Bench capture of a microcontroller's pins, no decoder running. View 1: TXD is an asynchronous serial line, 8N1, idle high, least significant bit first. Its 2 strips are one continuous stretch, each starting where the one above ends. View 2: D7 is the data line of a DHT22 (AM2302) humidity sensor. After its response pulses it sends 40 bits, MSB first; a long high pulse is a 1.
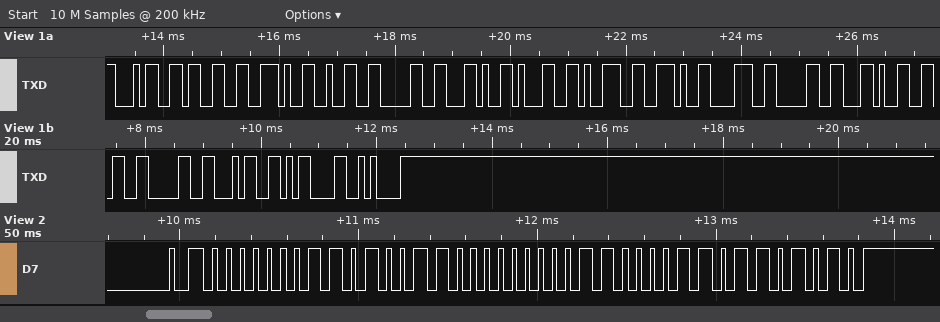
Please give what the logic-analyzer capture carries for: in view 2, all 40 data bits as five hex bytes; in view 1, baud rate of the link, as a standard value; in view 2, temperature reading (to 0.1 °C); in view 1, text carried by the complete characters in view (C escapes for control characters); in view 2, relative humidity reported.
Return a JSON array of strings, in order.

["01 A6 00 C3 6A", "9600 baud", "19.5 °C", "\"43.20,19.80,604\\r\\n\"", "42.2 %"]
